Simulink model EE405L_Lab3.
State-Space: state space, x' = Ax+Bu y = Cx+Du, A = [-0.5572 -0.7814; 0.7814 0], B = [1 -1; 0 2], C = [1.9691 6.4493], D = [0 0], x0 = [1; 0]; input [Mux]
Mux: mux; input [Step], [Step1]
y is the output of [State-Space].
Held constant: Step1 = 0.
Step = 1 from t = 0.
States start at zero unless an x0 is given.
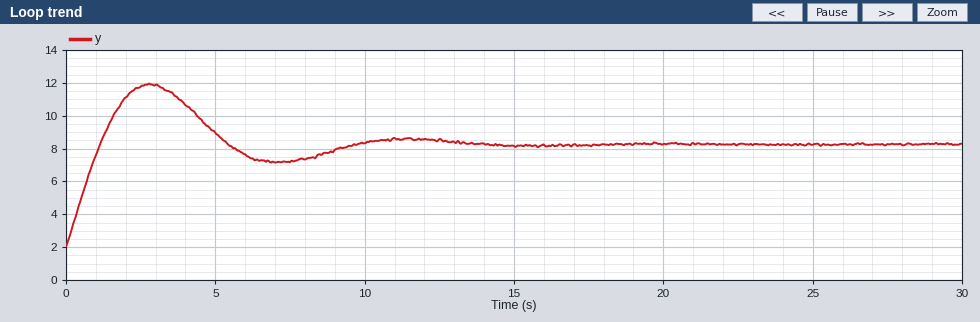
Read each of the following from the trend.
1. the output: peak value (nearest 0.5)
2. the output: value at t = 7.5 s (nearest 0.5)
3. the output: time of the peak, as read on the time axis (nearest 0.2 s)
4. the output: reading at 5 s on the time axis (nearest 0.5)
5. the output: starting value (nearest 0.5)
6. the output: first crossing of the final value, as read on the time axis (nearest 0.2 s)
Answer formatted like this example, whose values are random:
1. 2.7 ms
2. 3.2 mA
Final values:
1. 12.0
2. 7.0
3. 2.8 s
4. 9.0
5. 2.0
6. 1.2 s
